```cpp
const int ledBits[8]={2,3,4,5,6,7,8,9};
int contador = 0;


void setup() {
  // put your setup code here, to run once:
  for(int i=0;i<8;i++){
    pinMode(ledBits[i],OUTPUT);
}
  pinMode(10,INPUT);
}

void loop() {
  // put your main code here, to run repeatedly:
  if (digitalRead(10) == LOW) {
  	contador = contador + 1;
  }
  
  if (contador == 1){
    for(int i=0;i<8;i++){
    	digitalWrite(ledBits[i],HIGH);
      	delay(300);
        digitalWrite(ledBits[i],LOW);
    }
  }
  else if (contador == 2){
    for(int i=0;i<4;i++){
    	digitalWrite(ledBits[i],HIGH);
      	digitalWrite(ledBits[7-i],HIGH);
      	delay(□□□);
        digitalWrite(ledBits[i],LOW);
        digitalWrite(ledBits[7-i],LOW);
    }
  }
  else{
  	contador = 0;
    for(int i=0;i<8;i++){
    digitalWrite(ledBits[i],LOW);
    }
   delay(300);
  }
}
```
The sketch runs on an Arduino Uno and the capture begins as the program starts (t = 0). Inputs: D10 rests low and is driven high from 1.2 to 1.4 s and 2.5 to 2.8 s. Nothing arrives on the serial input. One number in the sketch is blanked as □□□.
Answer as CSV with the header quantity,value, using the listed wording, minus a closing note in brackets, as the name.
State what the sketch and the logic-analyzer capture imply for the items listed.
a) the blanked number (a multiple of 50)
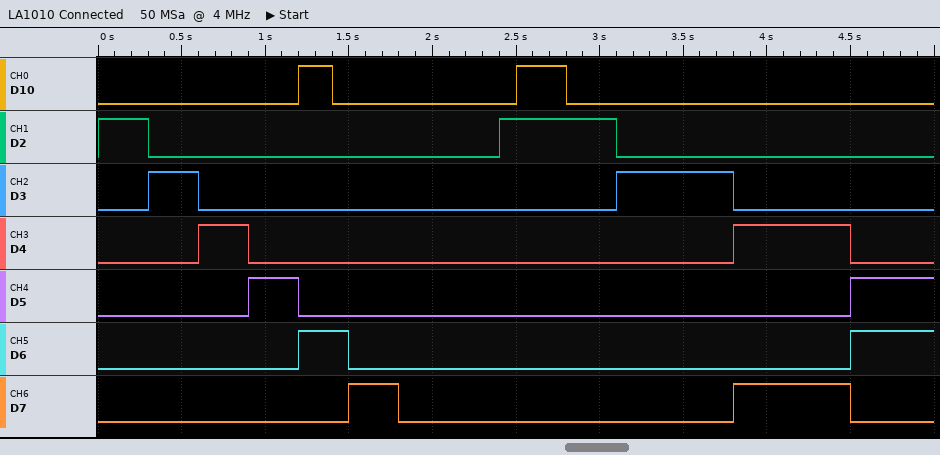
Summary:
quantity,value
the blanked number,700
